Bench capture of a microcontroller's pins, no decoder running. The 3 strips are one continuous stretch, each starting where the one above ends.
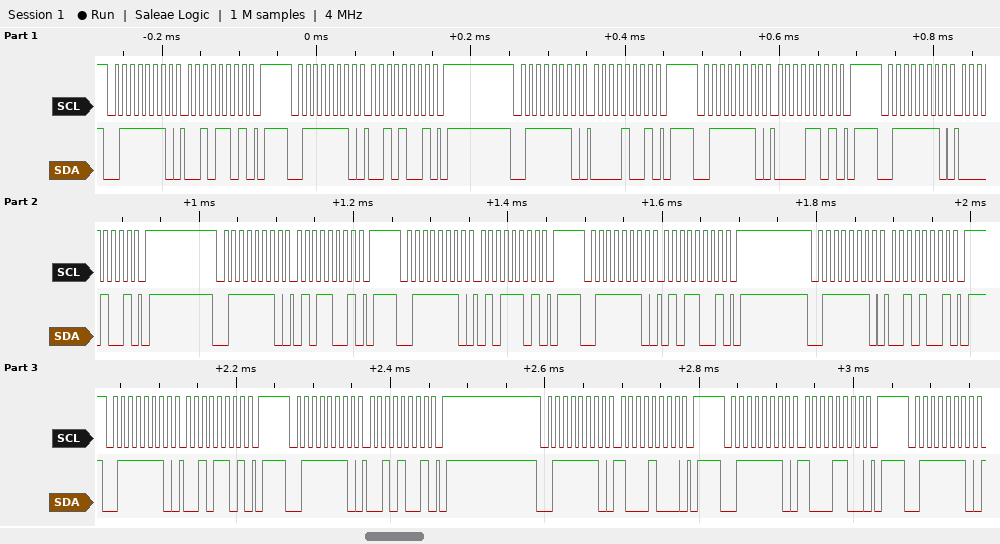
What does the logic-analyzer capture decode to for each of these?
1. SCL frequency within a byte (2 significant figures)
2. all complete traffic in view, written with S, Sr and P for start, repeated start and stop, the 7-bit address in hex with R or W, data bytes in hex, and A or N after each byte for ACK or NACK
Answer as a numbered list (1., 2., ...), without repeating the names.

1. 100 kHz
2. S 3FW A 2D A P S 3FW A 29 A P S 3FW A 09 A P S 3FW A 0D A P S 3FW A 09 A P S 3FW A 59 A P S 3FW A 5D A P S 3FW A 59 A P S 3FW A 29 A P S 3FW A 2D A P S 3FW A 29 A P S 3FW A 88 A P S 3FW A 8C A P S 3FW A
